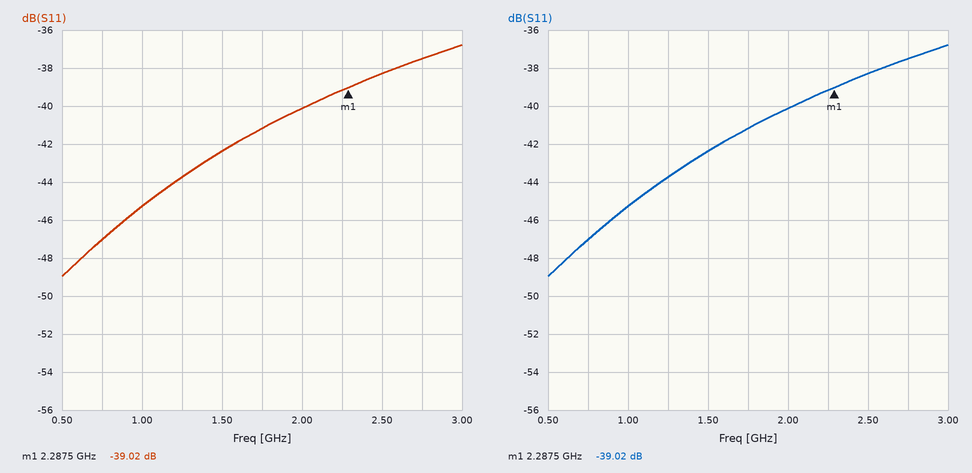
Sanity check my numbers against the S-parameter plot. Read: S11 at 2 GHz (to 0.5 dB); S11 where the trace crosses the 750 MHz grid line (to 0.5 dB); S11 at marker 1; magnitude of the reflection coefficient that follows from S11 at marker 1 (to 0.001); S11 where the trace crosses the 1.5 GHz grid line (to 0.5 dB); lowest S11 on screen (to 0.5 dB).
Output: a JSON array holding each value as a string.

["-40.0 dB", "-47.0 dB", "-39.02 dB", "0.011", "-42.5 dB", "-49.0 dB"]
